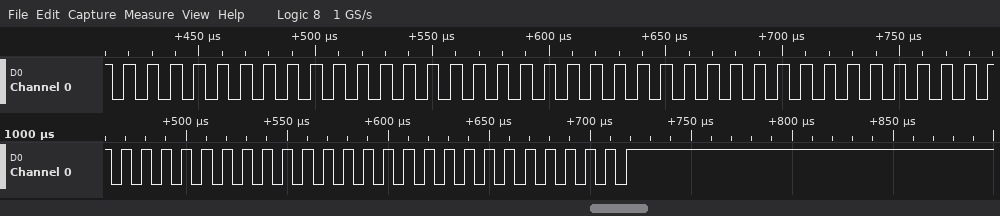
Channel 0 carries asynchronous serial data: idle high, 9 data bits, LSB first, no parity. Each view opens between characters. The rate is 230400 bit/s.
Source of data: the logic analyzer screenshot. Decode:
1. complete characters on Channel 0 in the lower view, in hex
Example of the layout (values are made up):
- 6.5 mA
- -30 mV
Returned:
- AD, AD, AD, AD, AD, 1FF
